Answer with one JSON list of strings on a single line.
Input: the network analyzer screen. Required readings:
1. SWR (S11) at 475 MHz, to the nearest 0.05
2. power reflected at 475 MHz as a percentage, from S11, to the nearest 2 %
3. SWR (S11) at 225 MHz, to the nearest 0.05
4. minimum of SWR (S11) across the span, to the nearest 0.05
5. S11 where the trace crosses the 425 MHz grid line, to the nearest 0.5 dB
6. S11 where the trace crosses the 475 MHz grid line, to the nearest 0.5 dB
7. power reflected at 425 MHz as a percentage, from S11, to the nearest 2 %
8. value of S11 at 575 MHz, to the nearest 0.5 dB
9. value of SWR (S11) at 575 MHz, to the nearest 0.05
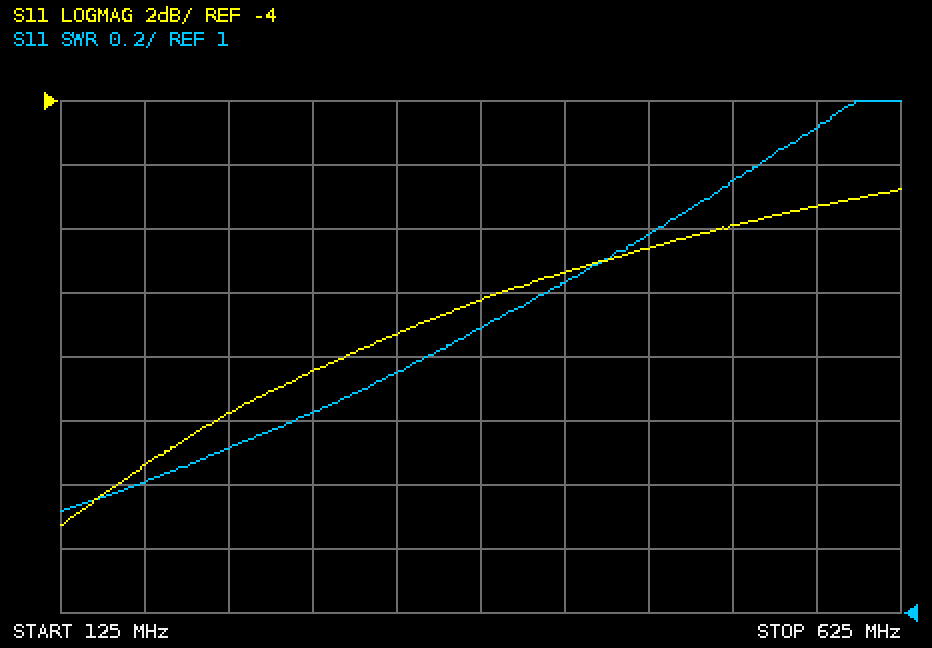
["2.20", "14 %", "1.50", "1.30", "-9.5 dB", "-8.5 dB", "12 %", "-7.5 dB", "2.50"]
